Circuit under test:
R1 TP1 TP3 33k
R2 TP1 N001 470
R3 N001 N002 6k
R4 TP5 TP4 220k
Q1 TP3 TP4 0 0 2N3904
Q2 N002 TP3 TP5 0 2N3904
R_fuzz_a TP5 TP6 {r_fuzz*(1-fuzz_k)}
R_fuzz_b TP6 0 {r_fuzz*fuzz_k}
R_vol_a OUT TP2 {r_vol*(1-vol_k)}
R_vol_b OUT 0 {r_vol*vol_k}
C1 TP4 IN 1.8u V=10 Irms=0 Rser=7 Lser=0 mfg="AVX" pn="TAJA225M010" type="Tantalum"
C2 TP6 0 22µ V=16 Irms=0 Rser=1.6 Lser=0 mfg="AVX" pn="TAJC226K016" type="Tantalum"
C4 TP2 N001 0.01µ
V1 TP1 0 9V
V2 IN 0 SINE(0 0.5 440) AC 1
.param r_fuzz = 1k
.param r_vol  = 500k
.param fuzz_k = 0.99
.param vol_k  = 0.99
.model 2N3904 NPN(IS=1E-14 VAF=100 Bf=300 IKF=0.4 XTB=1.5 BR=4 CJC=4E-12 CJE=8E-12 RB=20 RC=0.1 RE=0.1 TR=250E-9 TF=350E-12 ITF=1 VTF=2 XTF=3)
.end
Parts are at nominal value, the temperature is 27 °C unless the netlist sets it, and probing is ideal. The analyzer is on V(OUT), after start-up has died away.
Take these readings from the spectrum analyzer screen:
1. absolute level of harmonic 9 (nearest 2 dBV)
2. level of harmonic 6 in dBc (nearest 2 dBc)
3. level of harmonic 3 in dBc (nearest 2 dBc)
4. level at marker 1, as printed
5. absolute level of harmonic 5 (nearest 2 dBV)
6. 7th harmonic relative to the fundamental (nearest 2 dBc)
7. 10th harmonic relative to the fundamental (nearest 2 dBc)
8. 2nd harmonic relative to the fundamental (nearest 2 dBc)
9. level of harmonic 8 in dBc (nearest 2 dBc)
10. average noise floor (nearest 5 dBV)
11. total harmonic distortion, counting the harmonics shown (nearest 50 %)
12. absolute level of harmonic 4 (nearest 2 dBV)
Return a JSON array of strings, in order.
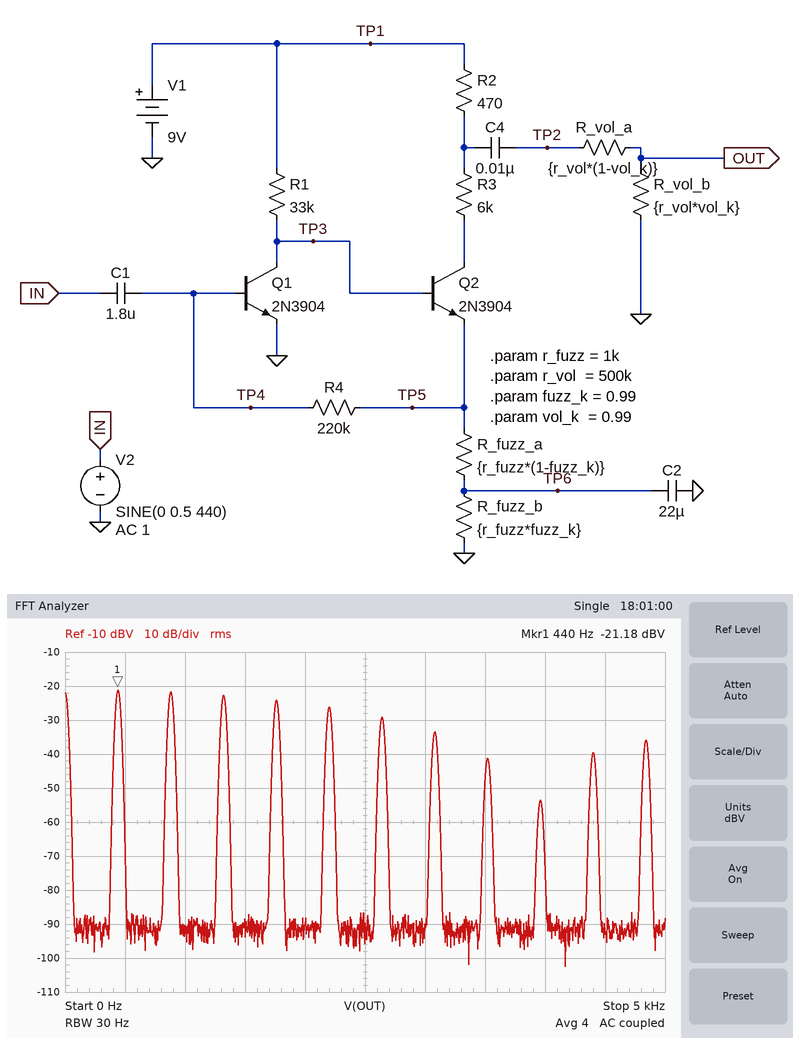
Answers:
["-54 dBV", "-8 dBc", "-2 dBc", "-21.18 dBV", "-26 dBV", "-12 dBc", "-18 dBc", "0 dBc", "-20 dBc", "-90 dBV", "150 %", "-24 dBV"]
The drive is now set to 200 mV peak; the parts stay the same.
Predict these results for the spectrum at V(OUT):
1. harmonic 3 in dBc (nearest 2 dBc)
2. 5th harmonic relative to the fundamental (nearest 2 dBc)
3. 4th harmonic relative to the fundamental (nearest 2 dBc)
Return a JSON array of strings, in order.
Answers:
["-2 dBc", "-10 dBc", "-6 dBc"]
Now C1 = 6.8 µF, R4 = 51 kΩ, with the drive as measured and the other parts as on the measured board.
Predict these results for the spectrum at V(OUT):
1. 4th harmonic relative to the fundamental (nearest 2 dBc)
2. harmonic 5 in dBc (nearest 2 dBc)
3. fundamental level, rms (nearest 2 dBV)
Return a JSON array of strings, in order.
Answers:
["-6 dBc", "-10 dBc", "-18 dBV"]
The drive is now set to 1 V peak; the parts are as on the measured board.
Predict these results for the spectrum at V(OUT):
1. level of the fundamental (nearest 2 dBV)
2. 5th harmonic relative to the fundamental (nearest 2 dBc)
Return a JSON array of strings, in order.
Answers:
["-22 dBV", "-4 dBc"]
